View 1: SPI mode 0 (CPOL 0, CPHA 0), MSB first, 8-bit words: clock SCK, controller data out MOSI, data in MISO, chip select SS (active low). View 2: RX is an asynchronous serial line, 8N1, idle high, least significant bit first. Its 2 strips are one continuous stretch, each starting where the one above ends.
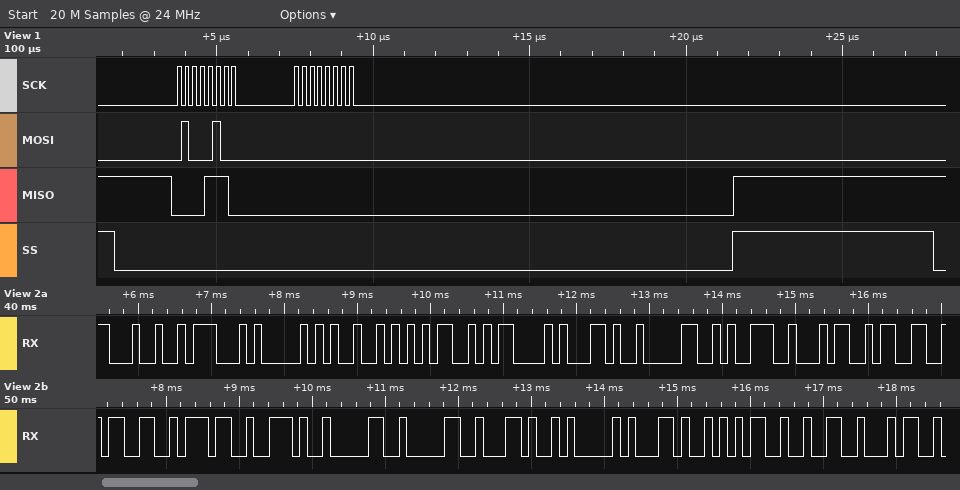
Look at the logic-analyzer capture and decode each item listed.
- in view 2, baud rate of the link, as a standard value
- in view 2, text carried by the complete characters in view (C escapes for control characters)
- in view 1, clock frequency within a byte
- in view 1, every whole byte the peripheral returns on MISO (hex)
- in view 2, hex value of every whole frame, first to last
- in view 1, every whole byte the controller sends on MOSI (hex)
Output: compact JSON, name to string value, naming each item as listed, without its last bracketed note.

{"in view 2, baud rate of the link, as a standard value": "9600 baud", "in view 2, text carried by the complete characters in view": "\"$GPRMC,094337.00,A,524\"", "in view 1, clock frequency within a byte": "4 MHz", "in view 1, every whole byte the peripheral returns on MISO": "0E 00", "in view 2, hex value of every whole frame, first to last": "24 47 50 52 4D 43 2C 30 39 34 33 33 37 2E 30 30 2C 41 2C 35 32 34", "in view 1, every whole byte the controller sends on MOSI": "44 00"}
